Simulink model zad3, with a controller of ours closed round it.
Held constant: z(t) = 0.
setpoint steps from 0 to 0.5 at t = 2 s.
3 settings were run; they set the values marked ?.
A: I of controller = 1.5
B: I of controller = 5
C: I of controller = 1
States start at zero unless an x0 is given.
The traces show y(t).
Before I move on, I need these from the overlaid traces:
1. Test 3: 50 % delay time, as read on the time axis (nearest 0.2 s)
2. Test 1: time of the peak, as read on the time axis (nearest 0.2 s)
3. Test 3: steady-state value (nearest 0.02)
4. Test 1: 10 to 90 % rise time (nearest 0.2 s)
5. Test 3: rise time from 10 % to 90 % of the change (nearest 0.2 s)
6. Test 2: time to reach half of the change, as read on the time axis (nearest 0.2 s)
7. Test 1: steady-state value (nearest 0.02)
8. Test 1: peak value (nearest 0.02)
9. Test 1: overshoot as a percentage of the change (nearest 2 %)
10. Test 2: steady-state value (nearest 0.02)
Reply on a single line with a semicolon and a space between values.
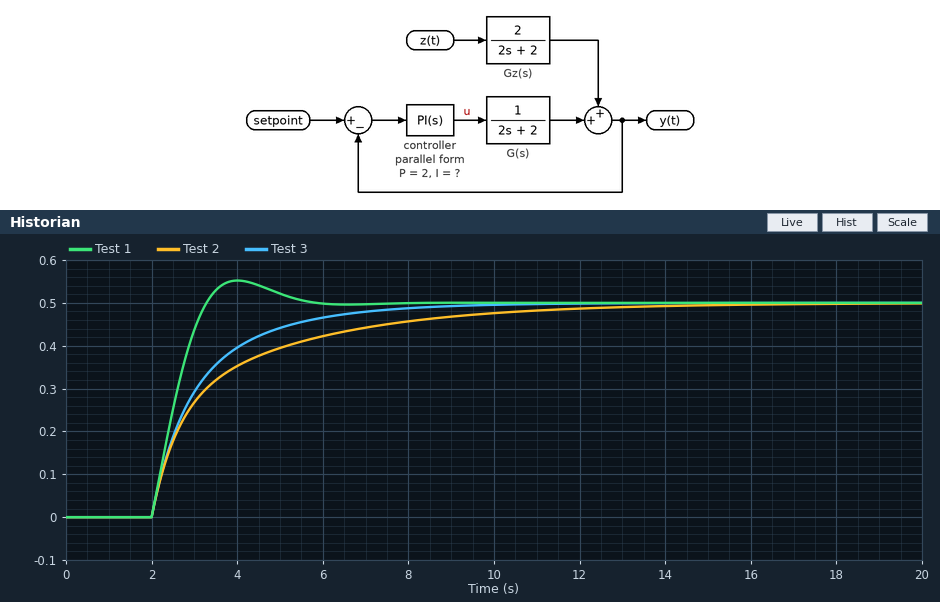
2.8 s; 4.0 s; 0.50; 1.0 s; 3.2 s; 2.8 s; 0.50; 0.56; 10 %; 0.50
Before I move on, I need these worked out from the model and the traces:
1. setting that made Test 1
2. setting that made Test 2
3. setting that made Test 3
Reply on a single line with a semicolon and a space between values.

B; C; A
